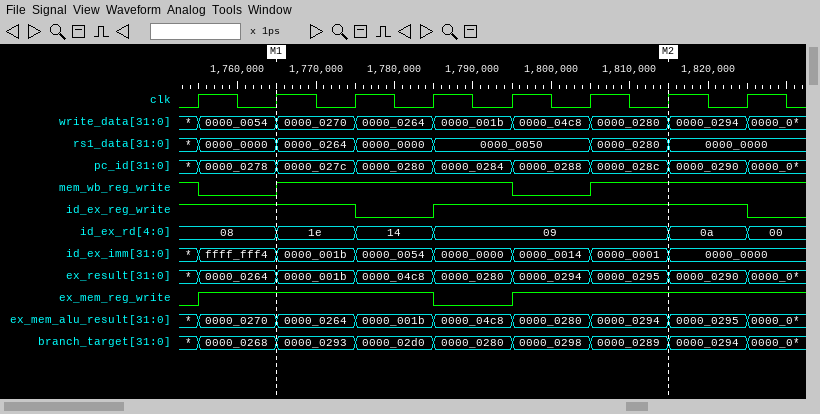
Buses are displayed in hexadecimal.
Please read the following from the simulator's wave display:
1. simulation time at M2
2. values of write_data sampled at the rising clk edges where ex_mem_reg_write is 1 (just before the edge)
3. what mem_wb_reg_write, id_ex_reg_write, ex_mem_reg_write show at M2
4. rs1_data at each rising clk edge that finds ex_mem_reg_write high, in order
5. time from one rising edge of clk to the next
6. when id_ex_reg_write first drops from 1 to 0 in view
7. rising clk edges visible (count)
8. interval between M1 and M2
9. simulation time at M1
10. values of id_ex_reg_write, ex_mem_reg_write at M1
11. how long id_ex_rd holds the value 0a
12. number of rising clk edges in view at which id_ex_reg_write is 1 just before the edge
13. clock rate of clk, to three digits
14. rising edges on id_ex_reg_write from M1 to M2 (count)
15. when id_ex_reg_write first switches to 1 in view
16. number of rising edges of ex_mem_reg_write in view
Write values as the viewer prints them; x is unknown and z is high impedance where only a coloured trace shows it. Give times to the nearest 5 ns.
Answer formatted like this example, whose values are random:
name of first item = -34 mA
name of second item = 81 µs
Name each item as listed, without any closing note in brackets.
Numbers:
simulation time at M2 = 1815 ns
values of write_data sampled at the rising clk edges where ex_mem_reg_write is 1 = 0000_0054, 0000_0270, 0000_0264, 0000_04c8, 0000_0280, 0000_0294
what mem_wb_reg_write, id_ex_reg_write, ex_mem_reg_write show at M2 = mem_wb_reg_write=1, id_ex_reg_write=1, ex_mem_reg_write=1
rs1_data at each rising clk edge that finds ex_mem_reg_write high, in order = 0000_0000, 0000_0264, 0000_0000, 0000_0050, 0000_0280, 0000_0000
time from one rising edge of clk to the next = 10 ns
when id_ex_reg_write first drops from 1 to 0 in view = 1775 ns
rising clk edges visible = 8
interval between M1 and M2 = 50 ns
simulation time at M1 = 1765 ns
values of id_ex_reg_write, ex_mem_reg_write at M1 = id_ex_reg_write=1, ex_mem_reg_write=1
how long id_ex_rd holds the value 0a = 10 ns
number of rising clk edges in view at which id_ex_reg_write is 1 just before the edge = 7
clock rate of clk, to three digits = 100 MHz
rising edges on id_ex_reg_write from M1 to M2 = 1
when id_ex_reg_write first switches to 1 in view = 1785 ns
number of rising edges of ex_mem_reg_write in view = 2
